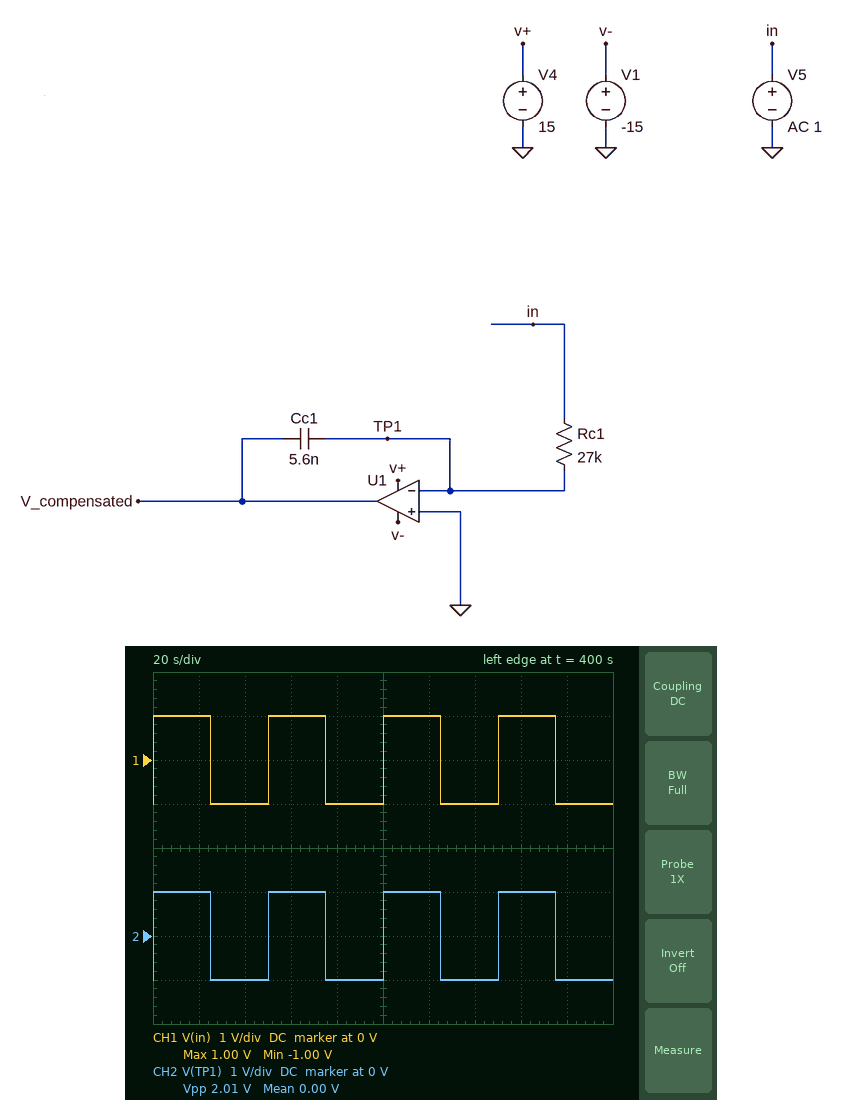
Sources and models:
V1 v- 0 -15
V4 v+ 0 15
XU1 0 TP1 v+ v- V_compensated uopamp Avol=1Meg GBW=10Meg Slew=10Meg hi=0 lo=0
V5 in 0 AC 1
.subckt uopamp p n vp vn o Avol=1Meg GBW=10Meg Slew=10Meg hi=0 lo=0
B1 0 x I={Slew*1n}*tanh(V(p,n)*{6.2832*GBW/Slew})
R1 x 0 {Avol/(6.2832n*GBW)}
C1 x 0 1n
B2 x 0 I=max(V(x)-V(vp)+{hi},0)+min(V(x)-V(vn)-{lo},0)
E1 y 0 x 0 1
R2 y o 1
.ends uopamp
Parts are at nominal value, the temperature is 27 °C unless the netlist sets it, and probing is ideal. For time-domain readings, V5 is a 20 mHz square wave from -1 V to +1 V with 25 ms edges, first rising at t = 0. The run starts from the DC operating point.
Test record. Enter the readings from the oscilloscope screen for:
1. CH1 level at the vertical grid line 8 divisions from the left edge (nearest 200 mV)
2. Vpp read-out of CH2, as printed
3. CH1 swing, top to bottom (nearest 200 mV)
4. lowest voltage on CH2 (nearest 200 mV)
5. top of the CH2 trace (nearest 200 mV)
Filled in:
1.0 V
2.01 V
2.0 V
-1.0 V
1.0 V
